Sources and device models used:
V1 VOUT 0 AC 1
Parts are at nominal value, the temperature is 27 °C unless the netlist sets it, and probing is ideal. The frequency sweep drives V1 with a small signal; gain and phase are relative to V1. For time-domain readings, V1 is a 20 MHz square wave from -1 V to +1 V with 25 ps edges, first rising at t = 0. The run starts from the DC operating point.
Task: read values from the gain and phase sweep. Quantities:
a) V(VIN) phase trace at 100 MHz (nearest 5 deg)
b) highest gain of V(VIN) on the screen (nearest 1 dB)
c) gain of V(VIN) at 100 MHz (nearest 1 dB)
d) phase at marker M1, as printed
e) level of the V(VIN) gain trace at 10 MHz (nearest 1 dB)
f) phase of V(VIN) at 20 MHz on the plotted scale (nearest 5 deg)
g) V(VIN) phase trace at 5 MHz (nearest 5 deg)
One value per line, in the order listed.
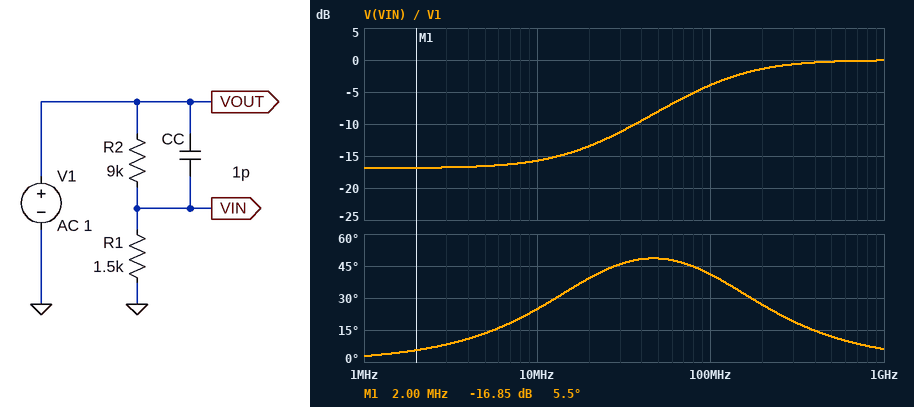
40 deg
0 dB
-4 dB
5.5 deg
-16 dB
40 deg
15 deg
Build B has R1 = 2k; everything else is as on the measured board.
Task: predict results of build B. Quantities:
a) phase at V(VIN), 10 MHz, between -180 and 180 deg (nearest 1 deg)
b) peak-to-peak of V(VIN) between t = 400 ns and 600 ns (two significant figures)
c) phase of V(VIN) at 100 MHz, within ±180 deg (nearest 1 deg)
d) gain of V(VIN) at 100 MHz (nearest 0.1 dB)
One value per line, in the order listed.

24 deg
3.6 V
34 deg
-2.8 dB
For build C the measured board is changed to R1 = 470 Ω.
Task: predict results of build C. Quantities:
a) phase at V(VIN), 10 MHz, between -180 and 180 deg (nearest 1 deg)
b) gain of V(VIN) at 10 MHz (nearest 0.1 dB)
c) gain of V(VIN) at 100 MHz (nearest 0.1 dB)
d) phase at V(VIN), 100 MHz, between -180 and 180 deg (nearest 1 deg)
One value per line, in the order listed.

28 deg
-24.9 dB
-11.2 dB
64 deg
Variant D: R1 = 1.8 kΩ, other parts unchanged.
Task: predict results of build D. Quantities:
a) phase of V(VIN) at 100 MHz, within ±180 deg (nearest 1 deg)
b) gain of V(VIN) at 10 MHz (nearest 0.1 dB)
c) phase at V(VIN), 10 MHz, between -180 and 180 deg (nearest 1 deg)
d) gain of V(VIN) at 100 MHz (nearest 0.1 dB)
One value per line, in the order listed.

37 deg
-14.4 dB
24 deg
-3.1 dB
